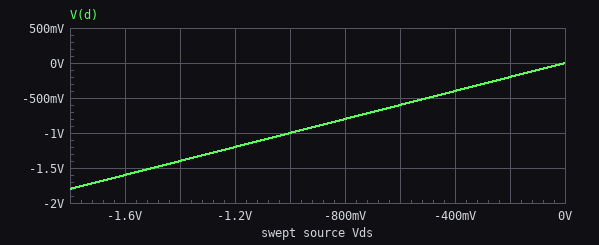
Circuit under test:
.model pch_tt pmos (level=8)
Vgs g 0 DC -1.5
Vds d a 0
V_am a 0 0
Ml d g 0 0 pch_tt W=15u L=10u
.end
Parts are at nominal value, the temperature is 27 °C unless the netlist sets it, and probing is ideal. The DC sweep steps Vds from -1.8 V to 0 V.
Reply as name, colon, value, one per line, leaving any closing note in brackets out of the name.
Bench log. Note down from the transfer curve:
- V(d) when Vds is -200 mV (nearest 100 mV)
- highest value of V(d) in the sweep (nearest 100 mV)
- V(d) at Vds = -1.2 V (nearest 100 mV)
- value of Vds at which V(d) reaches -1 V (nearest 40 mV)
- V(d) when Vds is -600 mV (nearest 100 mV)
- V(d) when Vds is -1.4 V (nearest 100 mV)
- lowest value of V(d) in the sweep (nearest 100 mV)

V(d) when Vds is -200 mV: -200 mV
highest value of V(d) in the sweep: 0 V
V(d) at Vds = -1.2 V: -1.2 V
value of Vds at which V(d) reaches -1 V: -1.00 V
V(d) when Vds is -600 mV: -600 mV
V(d) when Vds is -1.4 V: -1.4 V
lowest value of V(d) in the sweep: -1.8 V
